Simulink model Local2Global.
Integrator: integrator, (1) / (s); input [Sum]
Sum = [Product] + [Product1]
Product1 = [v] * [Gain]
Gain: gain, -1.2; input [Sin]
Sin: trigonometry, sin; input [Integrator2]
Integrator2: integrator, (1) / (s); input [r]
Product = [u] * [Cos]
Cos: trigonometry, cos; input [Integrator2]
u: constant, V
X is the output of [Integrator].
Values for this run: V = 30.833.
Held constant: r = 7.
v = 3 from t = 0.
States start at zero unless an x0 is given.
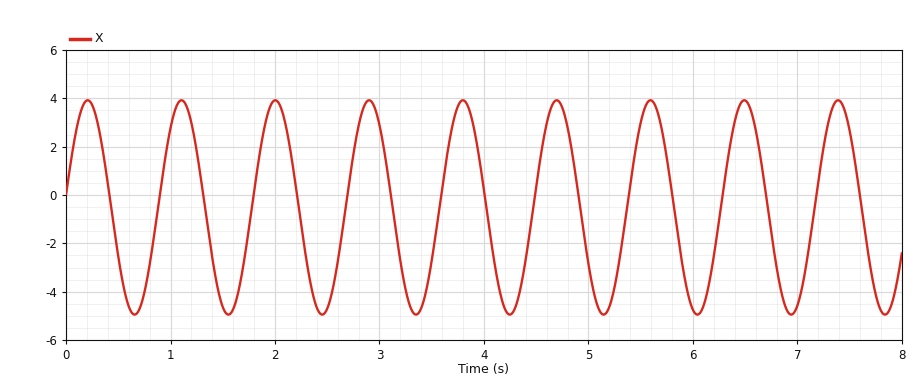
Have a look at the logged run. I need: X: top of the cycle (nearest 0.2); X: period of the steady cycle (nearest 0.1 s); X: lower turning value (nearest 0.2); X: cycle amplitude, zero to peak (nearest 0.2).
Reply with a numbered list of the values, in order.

1. 4.0
2. 0.9 s
3. -5.0
4. 4.4
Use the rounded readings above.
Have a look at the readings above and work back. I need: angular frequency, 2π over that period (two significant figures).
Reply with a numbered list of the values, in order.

1. 7.0 rad/s
